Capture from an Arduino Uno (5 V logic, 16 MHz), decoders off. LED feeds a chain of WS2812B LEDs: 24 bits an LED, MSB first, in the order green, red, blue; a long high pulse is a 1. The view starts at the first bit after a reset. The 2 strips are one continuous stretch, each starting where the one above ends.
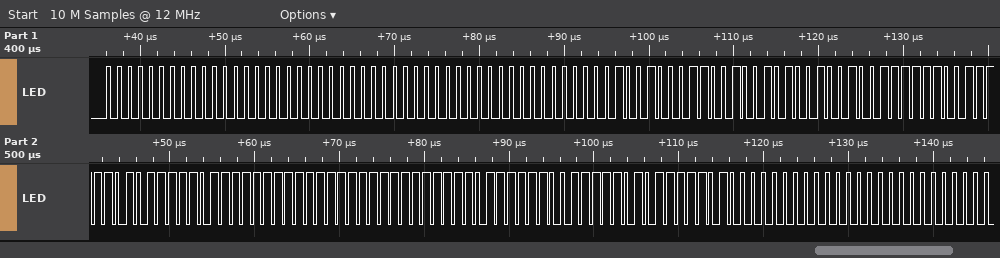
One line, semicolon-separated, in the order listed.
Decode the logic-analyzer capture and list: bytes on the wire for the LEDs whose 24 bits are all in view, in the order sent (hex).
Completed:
00 00 00 00 00 00 91 92 92 7E 7D 7D FF FF FF 7E 7D 7D 00 00 00
